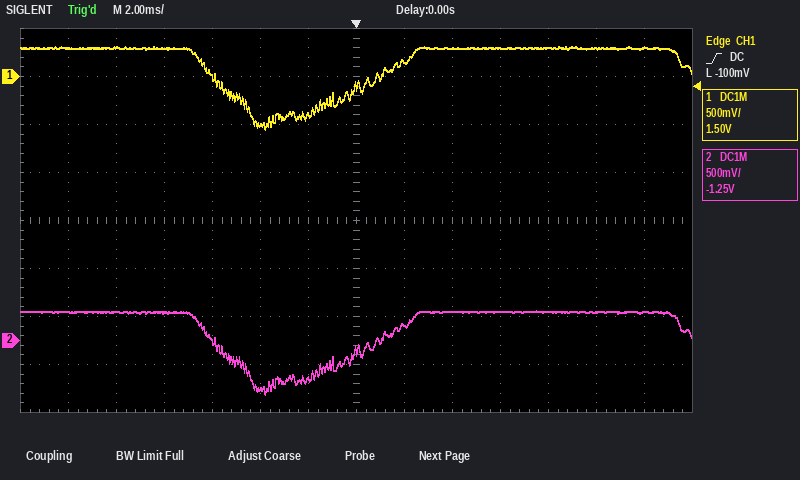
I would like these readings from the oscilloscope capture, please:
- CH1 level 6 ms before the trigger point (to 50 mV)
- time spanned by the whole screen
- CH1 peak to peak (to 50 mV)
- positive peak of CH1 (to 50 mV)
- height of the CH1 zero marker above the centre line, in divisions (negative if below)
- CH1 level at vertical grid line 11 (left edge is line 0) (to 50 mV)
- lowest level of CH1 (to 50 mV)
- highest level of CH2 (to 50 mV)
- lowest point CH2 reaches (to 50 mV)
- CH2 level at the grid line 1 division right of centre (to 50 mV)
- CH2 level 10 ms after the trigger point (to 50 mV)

0 mV
28 ms
850 mV
300 mV
+3.0 div
300 mV
-550 mV
300 mV
-550 mV
150 mV
300 mV
